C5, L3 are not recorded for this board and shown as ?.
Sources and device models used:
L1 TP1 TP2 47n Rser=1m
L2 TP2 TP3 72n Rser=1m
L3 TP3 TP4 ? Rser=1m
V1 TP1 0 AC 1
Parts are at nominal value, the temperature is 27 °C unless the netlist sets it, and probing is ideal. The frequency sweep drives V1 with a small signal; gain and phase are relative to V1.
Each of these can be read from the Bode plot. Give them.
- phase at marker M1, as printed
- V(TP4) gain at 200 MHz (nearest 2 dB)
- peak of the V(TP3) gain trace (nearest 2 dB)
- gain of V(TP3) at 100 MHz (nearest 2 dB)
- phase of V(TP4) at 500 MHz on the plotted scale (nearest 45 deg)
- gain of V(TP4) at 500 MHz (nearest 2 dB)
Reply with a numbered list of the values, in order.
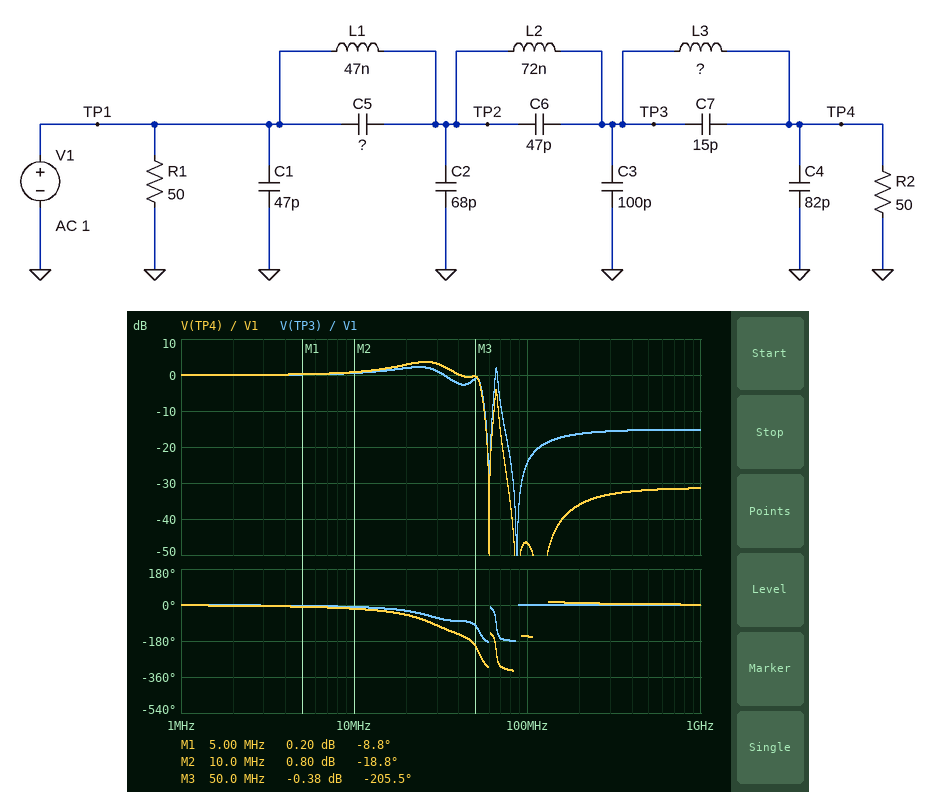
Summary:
1. -8.8 deg
2. -36 dB
3. 2 dB
4. -24 dB
5. 0 deg
6. -32 dB
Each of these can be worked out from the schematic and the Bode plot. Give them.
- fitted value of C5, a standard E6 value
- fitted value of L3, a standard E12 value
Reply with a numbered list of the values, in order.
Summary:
1. 150 pF
2. 120 nH
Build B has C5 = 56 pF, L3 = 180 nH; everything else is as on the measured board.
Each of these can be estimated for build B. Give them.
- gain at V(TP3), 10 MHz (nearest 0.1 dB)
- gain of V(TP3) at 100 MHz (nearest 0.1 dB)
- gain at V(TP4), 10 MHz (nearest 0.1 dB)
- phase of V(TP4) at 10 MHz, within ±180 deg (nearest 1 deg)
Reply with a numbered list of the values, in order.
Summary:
1. 0.4 dB
2. -51.3 dB
3. 0.7 dB
4. -23 deg
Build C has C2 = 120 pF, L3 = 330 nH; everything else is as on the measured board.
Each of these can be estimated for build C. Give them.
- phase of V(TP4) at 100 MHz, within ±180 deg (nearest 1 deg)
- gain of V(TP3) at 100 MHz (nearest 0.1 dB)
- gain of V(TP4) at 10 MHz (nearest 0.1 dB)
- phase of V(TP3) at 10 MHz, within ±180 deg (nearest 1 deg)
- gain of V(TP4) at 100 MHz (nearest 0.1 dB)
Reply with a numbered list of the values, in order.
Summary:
1. 20 deg
2. -27.5 dB
3. 0.4 dB
4. -9 deg
5. -49.7 dB
